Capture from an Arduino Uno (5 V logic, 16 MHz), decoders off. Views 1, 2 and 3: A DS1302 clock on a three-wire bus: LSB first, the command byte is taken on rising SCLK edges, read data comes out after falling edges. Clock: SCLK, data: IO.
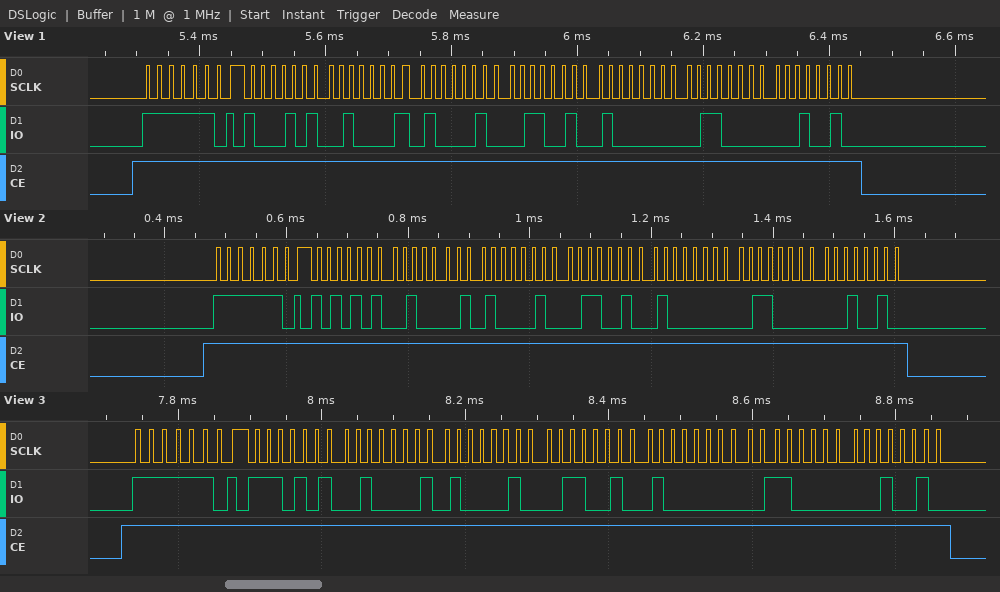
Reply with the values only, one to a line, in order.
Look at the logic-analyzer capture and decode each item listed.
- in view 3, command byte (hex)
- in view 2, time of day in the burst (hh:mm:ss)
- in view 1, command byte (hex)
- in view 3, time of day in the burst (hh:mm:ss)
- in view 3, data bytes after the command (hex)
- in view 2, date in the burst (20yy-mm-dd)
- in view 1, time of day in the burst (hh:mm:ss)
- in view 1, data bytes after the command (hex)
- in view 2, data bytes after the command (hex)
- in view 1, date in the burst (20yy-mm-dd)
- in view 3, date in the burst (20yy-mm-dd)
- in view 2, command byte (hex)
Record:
0xBF
21:42:55
0xBF
21:42:57
57 42 21 26 01 06 24
2024-01-26
21:42:51
51 42 21 26 01 06 24
55 42 21 26 01 06 24
2024-01-26
2024-01-26
0xBF
